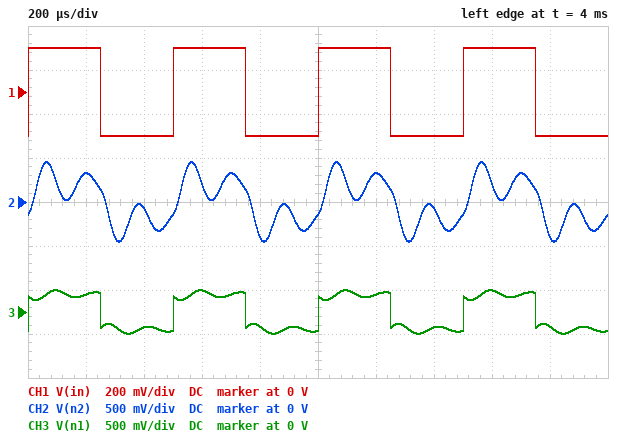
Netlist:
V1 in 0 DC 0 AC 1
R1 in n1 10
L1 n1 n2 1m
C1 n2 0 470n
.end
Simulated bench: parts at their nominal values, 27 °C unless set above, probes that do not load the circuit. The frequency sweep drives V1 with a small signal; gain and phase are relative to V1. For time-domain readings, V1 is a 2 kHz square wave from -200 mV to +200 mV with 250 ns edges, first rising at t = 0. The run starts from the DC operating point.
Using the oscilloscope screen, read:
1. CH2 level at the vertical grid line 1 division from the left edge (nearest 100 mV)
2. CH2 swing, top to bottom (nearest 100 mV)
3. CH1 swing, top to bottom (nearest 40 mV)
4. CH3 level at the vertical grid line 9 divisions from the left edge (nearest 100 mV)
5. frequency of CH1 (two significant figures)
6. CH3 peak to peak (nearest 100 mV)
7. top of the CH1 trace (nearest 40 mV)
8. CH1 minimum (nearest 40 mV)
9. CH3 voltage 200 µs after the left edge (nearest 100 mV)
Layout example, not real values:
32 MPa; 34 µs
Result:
300 mV; 900 mV; 400 mV; -200 mV; 2.0 kHz; 500 mV; 200 mV; -200 mV; 200 mV
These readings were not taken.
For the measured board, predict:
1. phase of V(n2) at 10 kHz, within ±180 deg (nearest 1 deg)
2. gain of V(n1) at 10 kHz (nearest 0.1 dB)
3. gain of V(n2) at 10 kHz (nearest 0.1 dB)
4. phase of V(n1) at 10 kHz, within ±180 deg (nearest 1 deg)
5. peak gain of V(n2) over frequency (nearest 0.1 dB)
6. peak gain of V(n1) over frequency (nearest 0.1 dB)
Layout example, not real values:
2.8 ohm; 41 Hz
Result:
-161 deg; -0.5 dB; 0.9 dB; 19 deg; 13.3 dB; 0 dB
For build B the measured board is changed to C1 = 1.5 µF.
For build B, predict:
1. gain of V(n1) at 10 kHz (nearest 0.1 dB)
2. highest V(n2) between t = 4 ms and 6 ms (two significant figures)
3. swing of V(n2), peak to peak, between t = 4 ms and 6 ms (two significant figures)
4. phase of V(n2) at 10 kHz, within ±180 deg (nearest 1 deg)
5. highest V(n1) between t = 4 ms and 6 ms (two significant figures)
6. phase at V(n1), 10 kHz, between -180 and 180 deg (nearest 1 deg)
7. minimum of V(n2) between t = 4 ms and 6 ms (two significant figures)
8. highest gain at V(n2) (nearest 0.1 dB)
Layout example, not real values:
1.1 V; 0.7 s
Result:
-0.2 dB; 370 mV; 730 mV; -169 deg; 250 mV; 11 deg; -370 mV; 8.4 dB
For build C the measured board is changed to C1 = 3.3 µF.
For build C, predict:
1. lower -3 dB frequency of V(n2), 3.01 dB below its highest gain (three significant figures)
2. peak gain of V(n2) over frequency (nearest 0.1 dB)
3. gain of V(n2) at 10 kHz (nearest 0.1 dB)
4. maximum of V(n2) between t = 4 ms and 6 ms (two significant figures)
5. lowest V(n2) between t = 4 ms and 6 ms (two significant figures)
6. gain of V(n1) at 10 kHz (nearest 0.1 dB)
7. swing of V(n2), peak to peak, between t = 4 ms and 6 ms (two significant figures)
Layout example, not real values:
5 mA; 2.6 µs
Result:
1.48 kHz; 5.2 dB; -21.7 dB; 390 mV; -390 mV; -0.1 dB; 780 mV
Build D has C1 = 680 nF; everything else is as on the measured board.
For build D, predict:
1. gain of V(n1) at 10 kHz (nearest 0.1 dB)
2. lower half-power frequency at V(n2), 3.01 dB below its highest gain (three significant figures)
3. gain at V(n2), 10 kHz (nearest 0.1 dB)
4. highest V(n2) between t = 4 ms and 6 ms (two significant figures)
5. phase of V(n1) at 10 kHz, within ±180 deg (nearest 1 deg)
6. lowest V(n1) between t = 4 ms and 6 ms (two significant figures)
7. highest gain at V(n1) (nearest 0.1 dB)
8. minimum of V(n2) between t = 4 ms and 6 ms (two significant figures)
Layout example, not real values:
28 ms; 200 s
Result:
-0.3 dB; 5.13 kHz; -4.8 dB; 570 mV; 14 deg; -280 mV; 0 dB; -570 mV
